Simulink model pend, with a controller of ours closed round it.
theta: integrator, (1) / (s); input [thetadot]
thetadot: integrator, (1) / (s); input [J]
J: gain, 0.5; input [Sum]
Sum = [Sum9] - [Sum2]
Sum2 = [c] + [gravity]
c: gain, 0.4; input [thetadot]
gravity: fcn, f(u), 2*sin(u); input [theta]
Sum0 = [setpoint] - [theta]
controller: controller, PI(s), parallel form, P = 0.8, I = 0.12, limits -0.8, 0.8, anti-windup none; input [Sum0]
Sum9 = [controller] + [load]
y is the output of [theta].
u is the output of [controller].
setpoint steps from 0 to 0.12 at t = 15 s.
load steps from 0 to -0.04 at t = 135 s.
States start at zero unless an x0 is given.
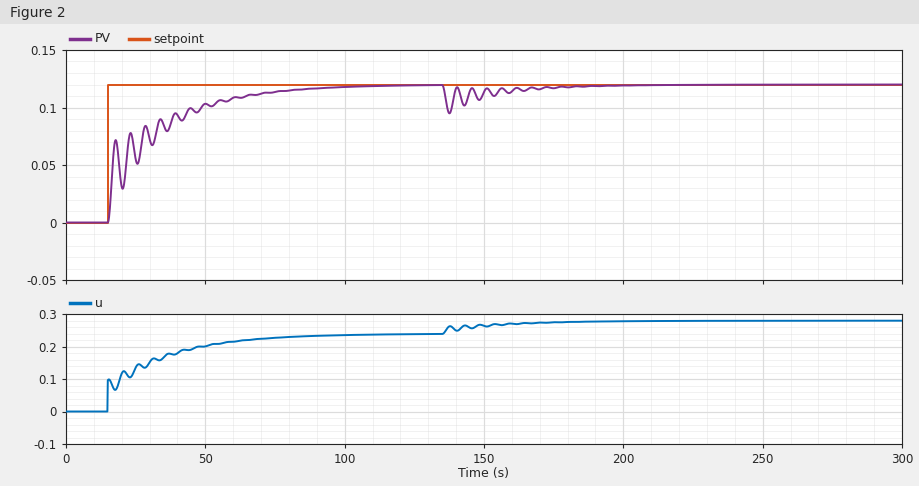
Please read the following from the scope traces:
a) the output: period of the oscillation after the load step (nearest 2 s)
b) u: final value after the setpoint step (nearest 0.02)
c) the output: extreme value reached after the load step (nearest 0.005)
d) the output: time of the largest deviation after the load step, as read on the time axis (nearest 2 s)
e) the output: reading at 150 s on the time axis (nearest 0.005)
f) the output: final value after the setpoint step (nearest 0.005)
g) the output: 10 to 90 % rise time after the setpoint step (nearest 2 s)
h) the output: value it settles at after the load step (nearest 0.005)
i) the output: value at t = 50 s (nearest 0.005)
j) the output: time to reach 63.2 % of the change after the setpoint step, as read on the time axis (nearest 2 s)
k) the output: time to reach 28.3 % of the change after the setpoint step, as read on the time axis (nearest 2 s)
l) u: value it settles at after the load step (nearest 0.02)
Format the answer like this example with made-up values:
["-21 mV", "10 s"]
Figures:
["6 s", "0.24", "0.095", "138 s", "0.115", "0.120", "44 s", "0.120", "0.105", "22 s", "16 s", "0.28"]
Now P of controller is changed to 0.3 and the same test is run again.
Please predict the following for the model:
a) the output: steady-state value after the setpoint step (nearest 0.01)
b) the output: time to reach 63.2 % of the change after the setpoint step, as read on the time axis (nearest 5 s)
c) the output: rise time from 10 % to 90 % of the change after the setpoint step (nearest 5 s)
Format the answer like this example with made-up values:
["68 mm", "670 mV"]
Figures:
["0.12", "30 s", "40 s"]
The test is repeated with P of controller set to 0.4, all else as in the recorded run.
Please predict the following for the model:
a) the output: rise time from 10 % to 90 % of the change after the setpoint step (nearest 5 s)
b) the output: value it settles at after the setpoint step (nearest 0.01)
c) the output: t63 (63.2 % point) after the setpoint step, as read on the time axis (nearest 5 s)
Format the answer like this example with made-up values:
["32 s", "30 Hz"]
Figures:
["40 s", "0.12", "30 s"]
